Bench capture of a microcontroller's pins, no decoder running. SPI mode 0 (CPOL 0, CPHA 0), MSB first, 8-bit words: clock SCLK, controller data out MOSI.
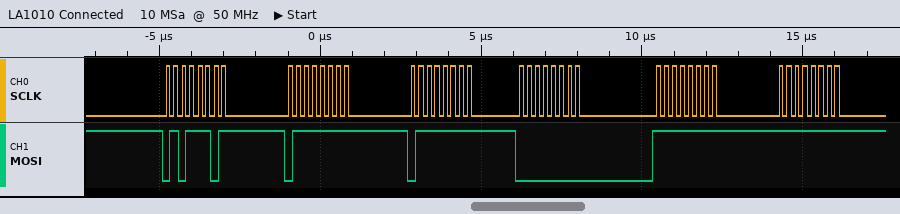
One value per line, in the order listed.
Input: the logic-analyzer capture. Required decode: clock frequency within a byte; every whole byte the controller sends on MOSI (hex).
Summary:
4 MHz
5D 7F 7F 00 FF FF
